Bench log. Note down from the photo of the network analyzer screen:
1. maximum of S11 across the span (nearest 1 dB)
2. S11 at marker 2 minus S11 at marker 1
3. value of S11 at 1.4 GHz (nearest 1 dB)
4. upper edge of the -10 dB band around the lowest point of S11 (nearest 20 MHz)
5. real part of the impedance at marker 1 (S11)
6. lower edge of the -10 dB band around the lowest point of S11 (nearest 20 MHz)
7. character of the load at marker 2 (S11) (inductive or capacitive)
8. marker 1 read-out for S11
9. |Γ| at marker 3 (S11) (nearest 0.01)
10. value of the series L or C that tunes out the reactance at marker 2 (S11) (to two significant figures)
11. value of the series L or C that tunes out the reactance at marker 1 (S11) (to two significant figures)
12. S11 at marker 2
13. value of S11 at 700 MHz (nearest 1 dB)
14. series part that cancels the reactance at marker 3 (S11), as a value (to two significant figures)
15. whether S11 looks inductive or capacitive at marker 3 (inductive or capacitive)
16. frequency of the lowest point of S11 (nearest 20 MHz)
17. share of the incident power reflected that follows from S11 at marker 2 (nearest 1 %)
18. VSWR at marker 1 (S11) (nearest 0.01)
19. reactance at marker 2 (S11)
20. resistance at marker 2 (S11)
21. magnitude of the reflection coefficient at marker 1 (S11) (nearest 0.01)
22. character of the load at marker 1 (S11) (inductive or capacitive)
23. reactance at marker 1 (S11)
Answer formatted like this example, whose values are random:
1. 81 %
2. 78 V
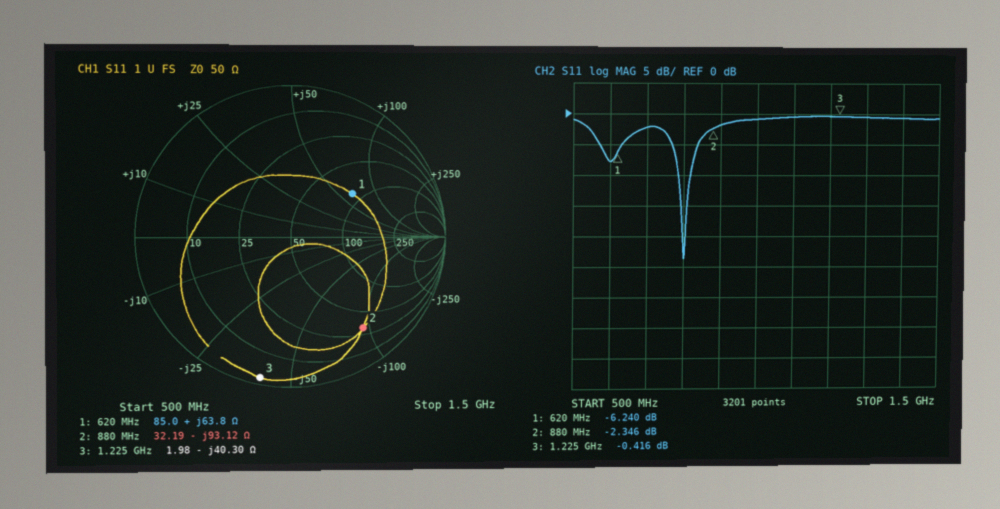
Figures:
1. 0 dB
2. 3.894 dB
3. -1 dB
4. 820 MHz
5. 85.0 Ω
6. 780 MHz
7. capacitive
8. -6.240 dB
9. 0.95
10. 17 nH
11. 4.0 pF
12. -2.346 dB
13. -2 dB
14. 5.2 nH
15. capacitive
16. 800 MHz
17. 58 %
18. 2.90
19. -93.12 Ω
20. 32.19 Ω
21. 0.49
22. inductive
23. +63.8 Ω
